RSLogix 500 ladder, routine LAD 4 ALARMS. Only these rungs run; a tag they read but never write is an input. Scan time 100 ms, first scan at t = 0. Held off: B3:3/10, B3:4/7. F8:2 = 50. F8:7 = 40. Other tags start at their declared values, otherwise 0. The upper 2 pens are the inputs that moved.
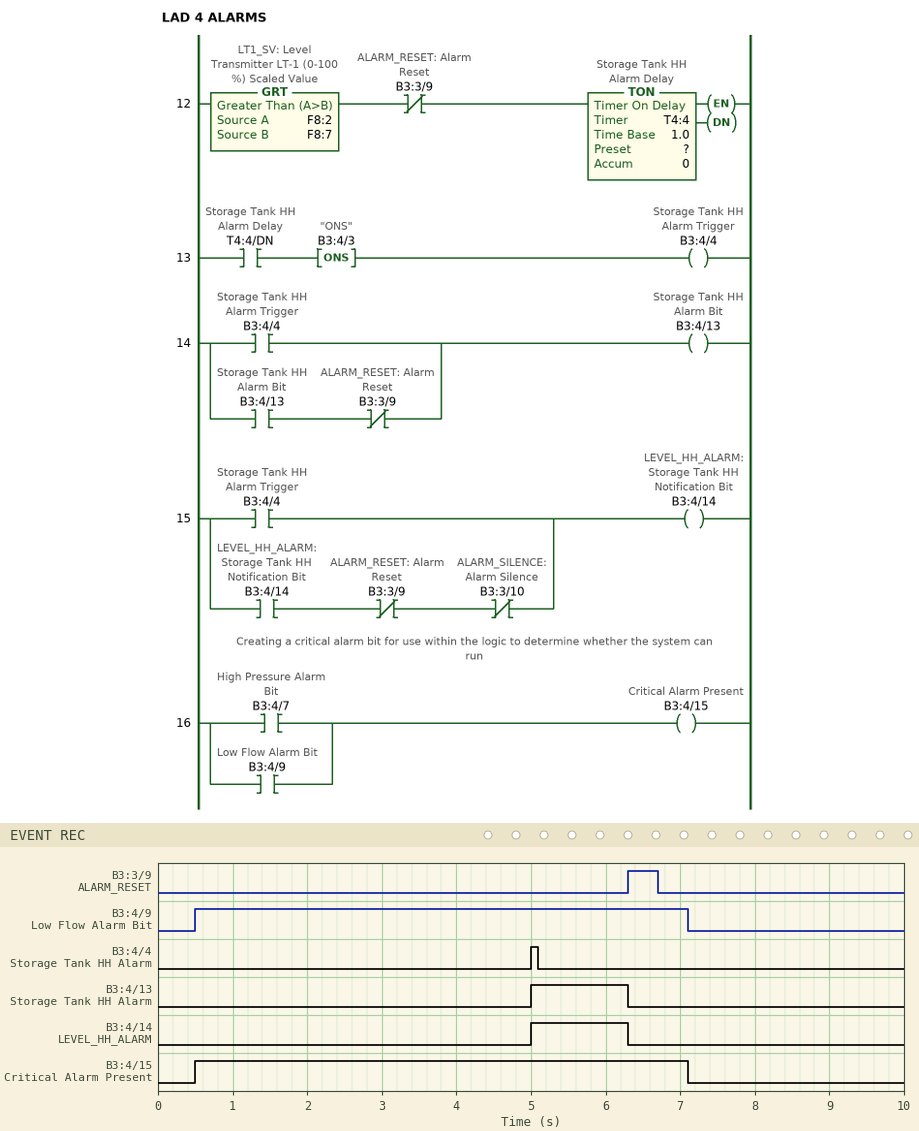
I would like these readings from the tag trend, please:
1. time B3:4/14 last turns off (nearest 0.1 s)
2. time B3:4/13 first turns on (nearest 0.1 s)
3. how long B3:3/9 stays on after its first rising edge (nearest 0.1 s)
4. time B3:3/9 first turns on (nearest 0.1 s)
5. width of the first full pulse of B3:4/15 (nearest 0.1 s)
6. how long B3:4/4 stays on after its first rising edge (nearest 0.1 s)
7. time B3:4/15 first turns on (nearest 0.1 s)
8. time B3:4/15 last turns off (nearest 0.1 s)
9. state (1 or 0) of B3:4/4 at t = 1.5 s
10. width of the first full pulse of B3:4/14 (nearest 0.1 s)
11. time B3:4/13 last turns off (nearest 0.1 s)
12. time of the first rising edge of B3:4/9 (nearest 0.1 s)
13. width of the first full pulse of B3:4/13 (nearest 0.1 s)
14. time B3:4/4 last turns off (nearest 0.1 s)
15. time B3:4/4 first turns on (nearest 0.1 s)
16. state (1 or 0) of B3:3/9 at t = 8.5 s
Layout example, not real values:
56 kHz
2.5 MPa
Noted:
6.3 s
5.0 s
0.4 s
6.3 s
6.6 s
0.1 s
0.5 s
7.1 s
0
1.3 s
6.3 s
0.5 s
1.3 s
5.1 s
5.0 s
0
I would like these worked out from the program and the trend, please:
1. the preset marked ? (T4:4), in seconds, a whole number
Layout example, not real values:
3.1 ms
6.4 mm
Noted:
5 s
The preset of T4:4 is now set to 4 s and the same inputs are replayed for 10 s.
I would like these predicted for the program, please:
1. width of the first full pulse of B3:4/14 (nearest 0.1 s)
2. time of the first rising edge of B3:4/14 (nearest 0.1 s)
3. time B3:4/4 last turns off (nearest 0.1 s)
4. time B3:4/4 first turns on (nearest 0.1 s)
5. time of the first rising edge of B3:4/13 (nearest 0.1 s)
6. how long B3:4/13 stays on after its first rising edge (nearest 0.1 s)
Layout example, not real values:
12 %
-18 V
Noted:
2.3 s
4.0 s
4.1 s
4.0 s
4.0 s
2.3 s
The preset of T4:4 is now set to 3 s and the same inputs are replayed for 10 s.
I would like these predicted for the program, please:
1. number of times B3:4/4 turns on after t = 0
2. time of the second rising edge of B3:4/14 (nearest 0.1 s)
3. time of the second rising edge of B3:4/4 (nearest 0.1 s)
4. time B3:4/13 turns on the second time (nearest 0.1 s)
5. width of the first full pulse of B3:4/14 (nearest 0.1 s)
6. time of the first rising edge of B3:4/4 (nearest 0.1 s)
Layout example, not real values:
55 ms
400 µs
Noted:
2
9.7 s
9.7 s
9.7 s
3.3 s
3.0 s
